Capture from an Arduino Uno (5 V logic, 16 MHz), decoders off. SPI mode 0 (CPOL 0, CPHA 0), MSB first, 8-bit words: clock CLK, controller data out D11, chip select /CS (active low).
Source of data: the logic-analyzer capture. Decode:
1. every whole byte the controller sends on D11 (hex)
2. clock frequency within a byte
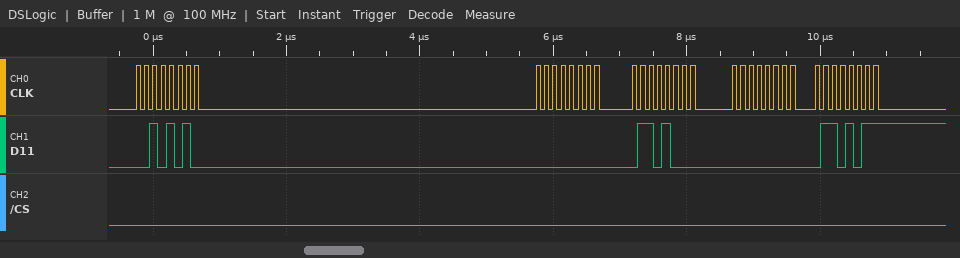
2A 00 68 00 6B
8 MHz
